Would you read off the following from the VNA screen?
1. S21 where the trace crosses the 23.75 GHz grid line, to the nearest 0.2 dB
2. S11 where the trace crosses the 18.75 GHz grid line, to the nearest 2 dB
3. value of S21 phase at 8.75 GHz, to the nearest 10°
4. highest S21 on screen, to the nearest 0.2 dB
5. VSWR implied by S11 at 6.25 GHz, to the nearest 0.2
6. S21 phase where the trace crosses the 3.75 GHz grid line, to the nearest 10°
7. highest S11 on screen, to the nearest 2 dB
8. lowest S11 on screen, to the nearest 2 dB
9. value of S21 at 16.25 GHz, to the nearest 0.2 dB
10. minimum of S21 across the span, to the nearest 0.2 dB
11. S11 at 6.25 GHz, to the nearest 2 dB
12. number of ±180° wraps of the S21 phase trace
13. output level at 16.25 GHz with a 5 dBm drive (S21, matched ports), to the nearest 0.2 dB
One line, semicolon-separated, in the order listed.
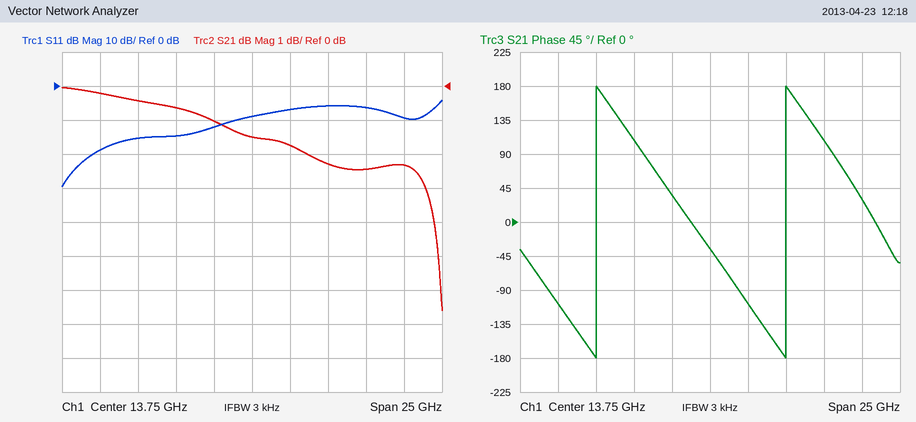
-2.4 dB; -6 dB; 110°; 0.0 dB; 1.4; -110°; -4 dB; -30 dB; -1.8 dB; -6.6 dB; -16 dB; 2; 3.2 dBm
